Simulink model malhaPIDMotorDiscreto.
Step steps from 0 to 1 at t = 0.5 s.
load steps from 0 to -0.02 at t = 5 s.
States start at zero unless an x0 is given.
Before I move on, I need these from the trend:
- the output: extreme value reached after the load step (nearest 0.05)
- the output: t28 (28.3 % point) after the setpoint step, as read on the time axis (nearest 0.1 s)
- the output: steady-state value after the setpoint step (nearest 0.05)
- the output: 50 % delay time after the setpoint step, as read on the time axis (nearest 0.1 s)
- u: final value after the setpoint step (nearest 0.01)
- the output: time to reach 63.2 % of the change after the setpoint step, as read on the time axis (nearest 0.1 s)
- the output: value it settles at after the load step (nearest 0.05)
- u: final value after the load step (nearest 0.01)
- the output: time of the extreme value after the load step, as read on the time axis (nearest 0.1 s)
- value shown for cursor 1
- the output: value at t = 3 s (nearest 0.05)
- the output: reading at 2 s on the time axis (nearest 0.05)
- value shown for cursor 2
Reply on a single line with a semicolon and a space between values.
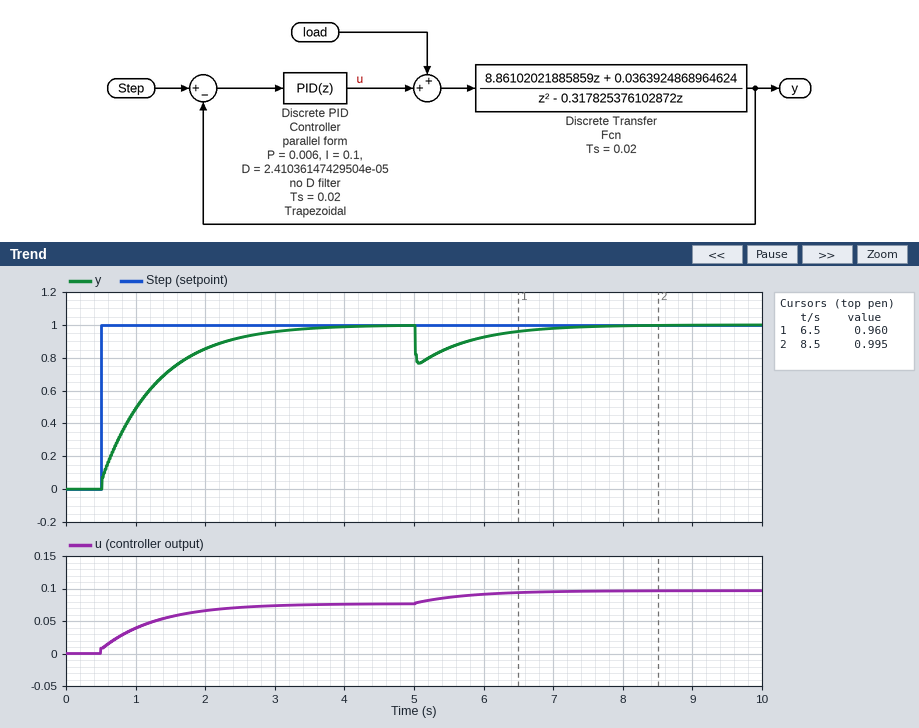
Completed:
0.75; 0.7 s; 1.00; 1.0 s; 0.08; 1.3 s; 1.00; 0.10; 5.1 s; 0.960; 0.95; 0.85; 0.995
